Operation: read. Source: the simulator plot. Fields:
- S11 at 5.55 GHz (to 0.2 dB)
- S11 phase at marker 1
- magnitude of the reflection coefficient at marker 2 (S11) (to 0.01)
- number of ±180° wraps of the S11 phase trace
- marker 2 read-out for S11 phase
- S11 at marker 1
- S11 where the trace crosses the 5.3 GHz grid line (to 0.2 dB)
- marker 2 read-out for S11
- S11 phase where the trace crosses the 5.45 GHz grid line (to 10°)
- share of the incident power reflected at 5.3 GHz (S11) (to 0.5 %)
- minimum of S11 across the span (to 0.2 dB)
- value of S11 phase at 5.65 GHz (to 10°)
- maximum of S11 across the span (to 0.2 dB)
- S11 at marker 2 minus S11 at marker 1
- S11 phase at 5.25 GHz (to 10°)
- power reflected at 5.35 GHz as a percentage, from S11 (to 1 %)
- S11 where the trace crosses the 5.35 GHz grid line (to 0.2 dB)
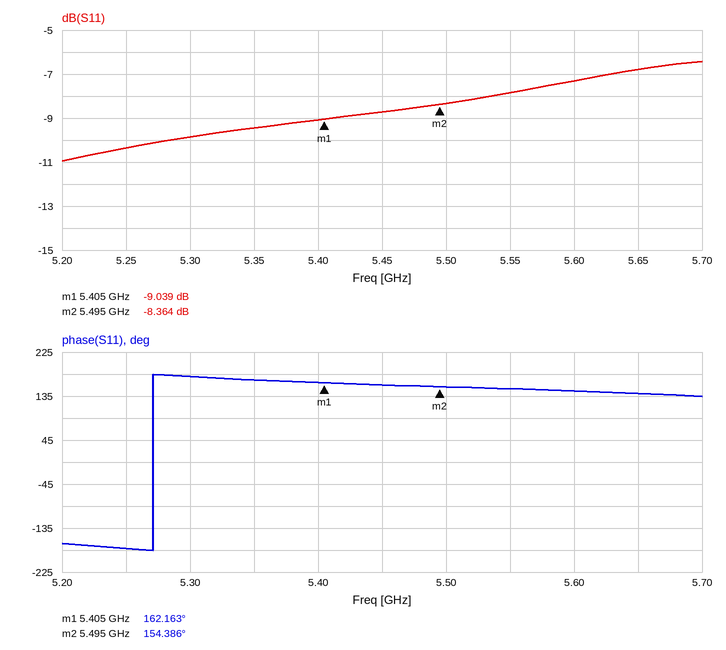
-7.8 dB
162.163°
0.38
1
154.386°
-9.039 dB
-9.8 dB
-8.364 dB
160°
10.5 %
-11.0 dB
140°
-6.4 dB
0.675 dB
-180°
11 %
-9.4 dB
